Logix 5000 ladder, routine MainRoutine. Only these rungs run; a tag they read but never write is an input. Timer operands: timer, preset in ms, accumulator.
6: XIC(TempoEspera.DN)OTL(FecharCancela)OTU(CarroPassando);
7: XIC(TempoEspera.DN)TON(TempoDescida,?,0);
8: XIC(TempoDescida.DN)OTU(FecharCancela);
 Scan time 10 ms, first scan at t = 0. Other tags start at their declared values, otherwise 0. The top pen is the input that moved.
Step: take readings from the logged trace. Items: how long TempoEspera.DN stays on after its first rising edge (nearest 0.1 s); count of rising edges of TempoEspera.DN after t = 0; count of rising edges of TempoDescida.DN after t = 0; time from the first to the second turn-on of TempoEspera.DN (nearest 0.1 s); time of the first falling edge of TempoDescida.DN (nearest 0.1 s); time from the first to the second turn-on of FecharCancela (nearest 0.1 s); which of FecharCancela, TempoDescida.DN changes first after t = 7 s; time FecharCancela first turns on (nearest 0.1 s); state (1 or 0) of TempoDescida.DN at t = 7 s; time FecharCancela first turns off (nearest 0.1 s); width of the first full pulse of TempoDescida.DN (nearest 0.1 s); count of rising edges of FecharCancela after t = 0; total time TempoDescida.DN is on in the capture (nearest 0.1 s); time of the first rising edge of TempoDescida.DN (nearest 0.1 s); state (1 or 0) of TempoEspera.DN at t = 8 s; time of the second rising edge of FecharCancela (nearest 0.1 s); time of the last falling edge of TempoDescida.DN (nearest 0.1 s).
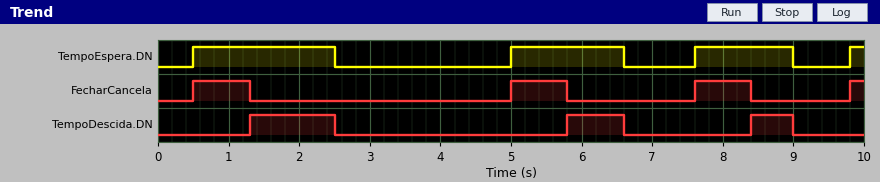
2.0 s
4
3
4.5 s
2.5 s
4.5 s
FecharCancela
0.5 s
0
1.3 s
1.2 s
4
2.6 s
1.3 s
1
5.0 s
9.0 s
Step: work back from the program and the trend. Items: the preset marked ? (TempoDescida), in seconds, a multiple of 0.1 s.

0.8 s
